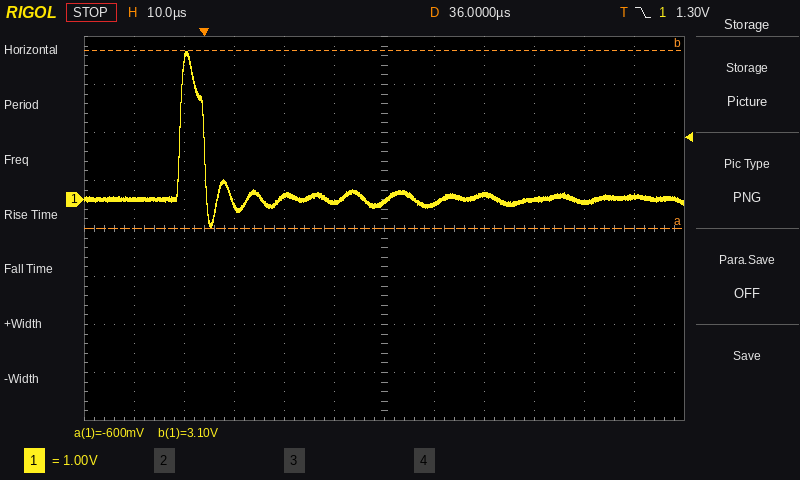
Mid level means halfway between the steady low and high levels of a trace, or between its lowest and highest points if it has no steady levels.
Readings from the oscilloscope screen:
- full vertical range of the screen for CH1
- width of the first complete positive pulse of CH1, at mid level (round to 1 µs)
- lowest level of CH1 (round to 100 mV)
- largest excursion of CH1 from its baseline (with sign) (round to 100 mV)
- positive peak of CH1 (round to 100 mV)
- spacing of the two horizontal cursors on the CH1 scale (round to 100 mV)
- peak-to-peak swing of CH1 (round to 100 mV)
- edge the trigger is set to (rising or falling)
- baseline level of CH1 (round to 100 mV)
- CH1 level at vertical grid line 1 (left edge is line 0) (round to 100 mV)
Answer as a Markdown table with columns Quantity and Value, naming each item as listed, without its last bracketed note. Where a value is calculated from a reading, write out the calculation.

| Quantity | Value |
|---|---|
| full vertical range of the screen for CH1 | 8 V |
| width of the first complete positive pulse of CH1, at mid level | 5 µs |
| lowest level of CH1 | -600 mV |
| largest excursion of CH1 from its baseline (with sign) | 3.1 V − (0.0 V) = +3.1 V |
| positive peak of CH1 | 3.1 V |
| spacing of the two horizontal cursors on the CH1 scale | 3.7 V |
| peak-to-peak swing of CH1 | 3.1 V − (-600 mV) = 3.7 V |
| edge the trigger is set to | falling |
| baseline level of CH1 | 0.0 V |
| CH1 level at vertical grid line 1 (left edge is line 0) | 0.0 V |
